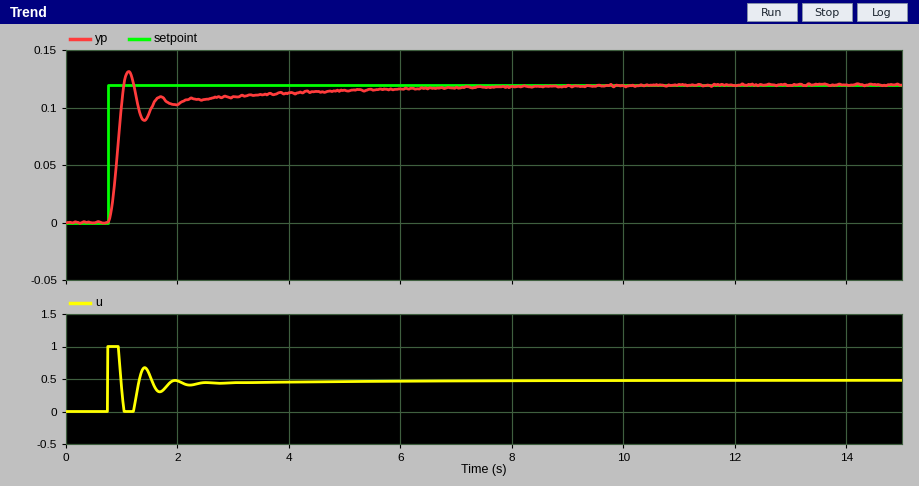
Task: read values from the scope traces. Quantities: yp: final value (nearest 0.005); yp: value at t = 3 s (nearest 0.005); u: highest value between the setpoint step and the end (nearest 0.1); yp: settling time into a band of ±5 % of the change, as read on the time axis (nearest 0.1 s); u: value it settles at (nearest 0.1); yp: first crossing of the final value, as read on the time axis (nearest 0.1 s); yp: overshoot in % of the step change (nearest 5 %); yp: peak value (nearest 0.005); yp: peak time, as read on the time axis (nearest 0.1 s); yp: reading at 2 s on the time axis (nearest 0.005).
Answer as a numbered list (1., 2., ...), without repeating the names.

1. 0.120
2. 0.110
3. 1.0
4. 4.7 s
5. 0.5
6. 1.0 s
7. 10 %
8. 0.130
9. 1.1 s
10. 0.105
